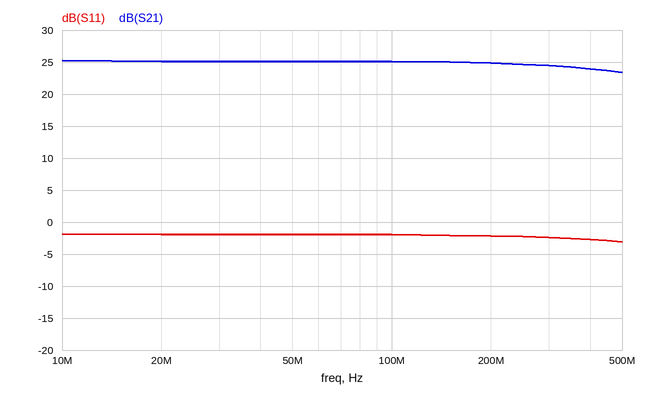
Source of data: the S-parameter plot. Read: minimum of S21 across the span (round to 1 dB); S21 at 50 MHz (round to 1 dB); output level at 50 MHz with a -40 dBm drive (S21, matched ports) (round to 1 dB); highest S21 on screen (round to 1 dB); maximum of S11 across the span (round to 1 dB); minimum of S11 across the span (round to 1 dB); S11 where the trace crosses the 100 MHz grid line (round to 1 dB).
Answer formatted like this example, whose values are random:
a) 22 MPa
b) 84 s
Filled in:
a) 23 dB
b) 25 dB
c) -15 dBm
d) 25 dB
e) -2 dB
f) -3 dB
g) -2 dB
